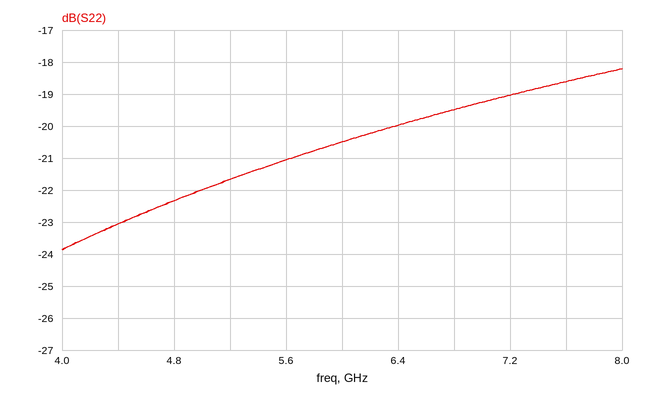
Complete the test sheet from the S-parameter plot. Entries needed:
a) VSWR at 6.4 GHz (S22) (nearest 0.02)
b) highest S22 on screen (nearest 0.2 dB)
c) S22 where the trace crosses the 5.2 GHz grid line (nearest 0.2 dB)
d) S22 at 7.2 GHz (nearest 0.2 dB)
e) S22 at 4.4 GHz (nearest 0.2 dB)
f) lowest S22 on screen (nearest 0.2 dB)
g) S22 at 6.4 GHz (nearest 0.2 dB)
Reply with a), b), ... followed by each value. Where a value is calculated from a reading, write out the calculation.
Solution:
a) |Γ| = 10^(-20/20) = 0.1000; VSWR = (1 + 0.1000)/(1 − 0.1000) ≈ 1.22
b) -18.2 dB
c) -21.6 dB
d) -19.0 dB
e) -23.0 dB
f) -23.8 dB
g) -20.0 dB
